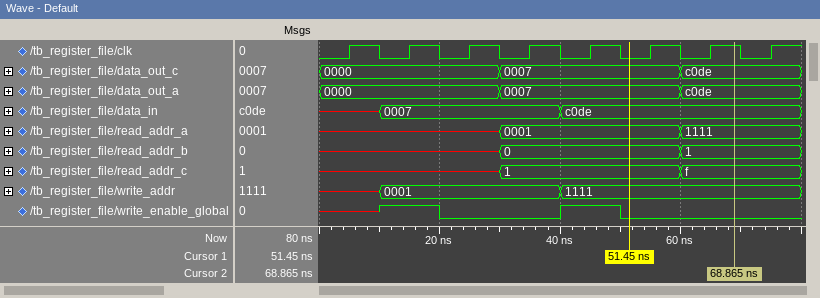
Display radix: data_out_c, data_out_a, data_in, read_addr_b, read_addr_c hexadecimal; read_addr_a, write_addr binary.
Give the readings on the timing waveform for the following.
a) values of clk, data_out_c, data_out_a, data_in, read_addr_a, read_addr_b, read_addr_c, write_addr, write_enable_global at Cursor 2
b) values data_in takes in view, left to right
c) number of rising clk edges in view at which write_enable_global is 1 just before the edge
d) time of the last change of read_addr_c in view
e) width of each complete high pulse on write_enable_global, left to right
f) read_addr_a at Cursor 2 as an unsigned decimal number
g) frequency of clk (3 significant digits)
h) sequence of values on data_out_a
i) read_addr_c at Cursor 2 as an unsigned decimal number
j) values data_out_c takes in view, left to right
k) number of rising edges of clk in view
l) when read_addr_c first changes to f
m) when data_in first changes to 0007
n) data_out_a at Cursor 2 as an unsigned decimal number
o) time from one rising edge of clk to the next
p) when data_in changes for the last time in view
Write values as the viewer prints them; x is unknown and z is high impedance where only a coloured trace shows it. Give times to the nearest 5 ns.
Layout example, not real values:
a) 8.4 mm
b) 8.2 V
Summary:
a) clk=1, data_out_c=c0de, data_out_a=c0de, data_in=c0de, read_addr_a=1111, read_addr_b=1, read_addr_c=f, write_addr=1111, write_enable_global=0
b) x, 0007, c0de
c) 2
d) 60 ns
e) 10 ns
f) 15
g) 100 MHz
h) 0000, 0007, c0de
i) 15
j) 0000, 0007, c0de
k) 8
l) 60 ns
m) 10 ns
n) 49374
o) 10 ns
p) 40 ns
